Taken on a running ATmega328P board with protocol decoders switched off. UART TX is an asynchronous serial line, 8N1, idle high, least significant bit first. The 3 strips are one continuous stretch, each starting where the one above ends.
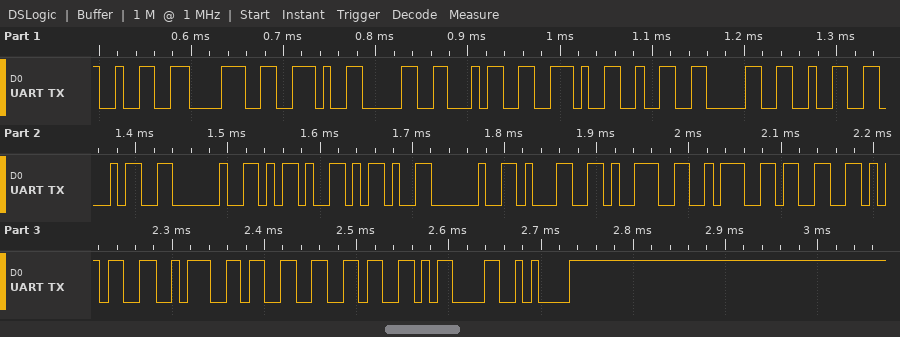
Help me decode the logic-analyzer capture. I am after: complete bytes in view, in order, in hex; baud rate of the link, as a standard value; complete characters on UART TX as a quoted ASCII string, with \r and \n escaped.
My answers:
32 38 2E 30 34 2E 32 30 32 34 20 2D 2D 20 31 39 3A 33 35 3A 33 36 0D 0A
115200 baud
"28.04.2024 -- 19:35:36\r\n"
